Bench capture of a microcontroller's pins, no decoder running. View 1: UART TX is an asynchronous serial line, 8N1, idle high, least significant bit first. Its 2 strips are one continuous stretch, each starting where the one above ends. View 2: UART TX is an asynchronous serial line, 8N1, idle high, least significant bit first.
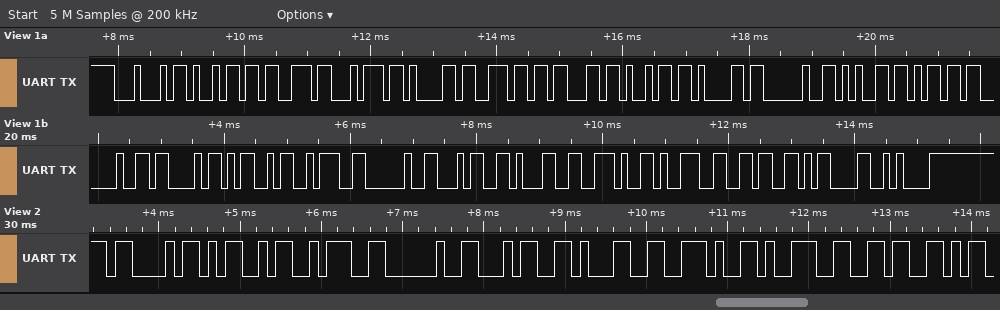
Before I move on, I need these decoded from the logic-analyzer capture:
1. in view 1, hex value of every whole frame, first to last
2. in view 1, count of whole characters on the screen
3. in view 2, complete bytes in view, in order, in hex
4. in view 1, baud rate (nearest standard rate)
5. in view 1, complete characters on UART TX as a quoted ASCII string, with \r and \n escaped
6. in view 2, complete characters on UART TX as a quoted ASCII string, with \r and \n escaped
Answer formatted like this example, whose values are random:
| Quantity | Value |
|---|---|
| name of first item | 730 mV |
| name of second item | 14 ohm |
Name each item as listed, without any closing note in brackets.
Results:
| Quantity | Value |
|---|---|
| in view 1, hex value of every whole frame, first to last | 44 69 73 74 61 6E 63 69 61 20 65 6D 20 43 4D 3A 20 34 31 2E 39 36 0D 0A |
| in view 1, count of whole characters on the screen | 24 |
| in view 2, complete bytes in view, in order, in hex | 43 4D 3A 20 34 31 2E 39 36 |
| in view 1, baud rate | 9600 baud |
| in view 1, complete characters on UART TX as a quoted ASCII string, with \r and \n escaped | "Distancia em CM: 41.96\r\n" |
| in view 2, complete characters on UART TX as a quoted ASCII string, with \r and \n escaped | "CM: 41.96" |
